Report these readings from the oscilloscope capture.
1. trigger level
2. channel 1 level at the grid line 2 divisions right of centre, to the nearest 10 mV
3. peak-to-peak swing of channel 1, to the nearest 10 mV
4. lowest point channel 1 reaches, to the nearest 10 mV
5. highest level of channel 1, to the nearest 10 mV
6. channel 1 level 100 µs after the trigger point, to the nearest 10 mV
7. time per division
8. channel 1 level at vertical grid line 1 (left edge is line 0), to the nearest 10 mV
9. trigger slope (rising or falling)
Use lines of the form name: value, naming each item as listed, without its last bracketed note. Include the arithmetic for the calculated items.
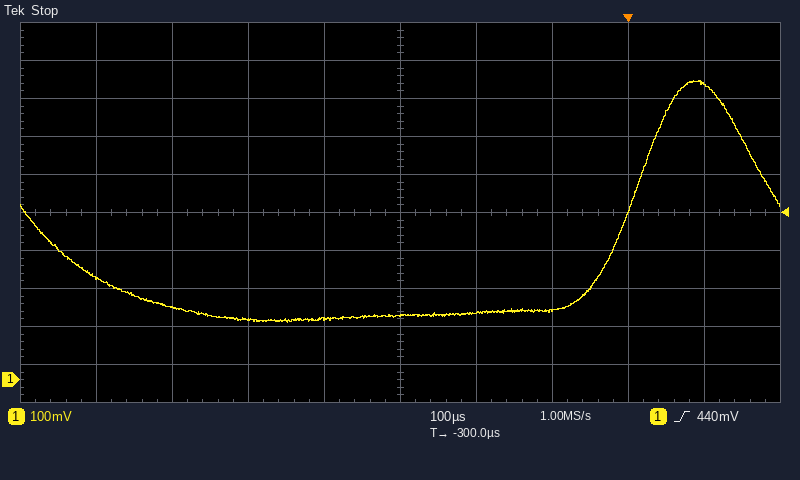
trigger level: 440 mV
channel 1 level at the grid line 2 divisions right of centre, to the nearest 10 mV: 180 mV
peak-to-peak swing of channel 1, to the nearest 10 mV: 790 mV − (150 mV) = 640 mV
lowest point channel 1 reaches, to the nearest 10 mV: 150 mV
highest level of channel 1, to the nearest 10 mV: 790 mV
channel 1 level 100 µs after the trigger point, to the nearest 10 mV: 780 mV
time per division: 100 µs
channel 1 level at vertical grid line 1 (left edge is line 0), to the nearest 10 mV: 270 mV
trigger slope: rising
